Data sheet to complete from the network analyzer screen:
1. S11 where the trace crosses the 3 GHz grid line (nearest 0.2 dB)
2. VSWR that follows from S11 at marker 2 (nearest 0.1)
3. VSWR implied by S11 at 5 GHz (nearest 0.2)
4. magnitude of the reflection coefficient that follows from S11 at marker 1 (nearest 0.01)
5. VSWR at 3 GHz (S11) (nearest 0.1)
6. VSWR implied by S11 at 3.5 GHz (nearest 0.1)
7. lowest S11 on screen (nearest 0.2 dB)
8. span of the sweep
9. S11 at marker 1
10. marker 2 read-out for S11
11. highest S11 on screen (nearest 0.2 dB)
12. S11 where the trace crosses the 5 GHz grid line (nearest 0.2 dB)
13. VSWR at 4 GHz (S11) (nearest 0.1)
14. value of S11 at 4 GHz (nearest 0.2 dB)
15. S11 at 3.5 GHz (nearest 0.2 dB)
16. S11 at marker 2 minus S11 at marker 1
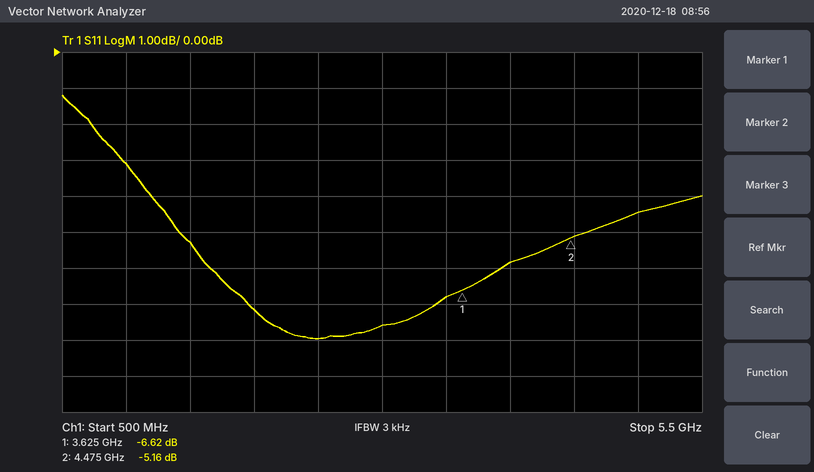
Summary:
-7.6 dB
3.5
4.0
0.47
2.4
2.7
-8.0 dB
5 GHz
-6.62 dB
-5.16 dB
-1.2 dB
-4.4 dB
3.1
-5.8 dB
-6.8 dB
1.46 dB
